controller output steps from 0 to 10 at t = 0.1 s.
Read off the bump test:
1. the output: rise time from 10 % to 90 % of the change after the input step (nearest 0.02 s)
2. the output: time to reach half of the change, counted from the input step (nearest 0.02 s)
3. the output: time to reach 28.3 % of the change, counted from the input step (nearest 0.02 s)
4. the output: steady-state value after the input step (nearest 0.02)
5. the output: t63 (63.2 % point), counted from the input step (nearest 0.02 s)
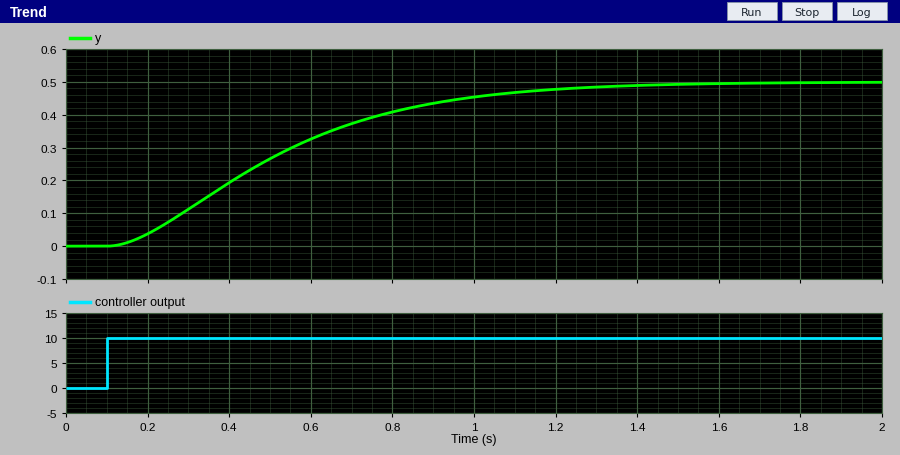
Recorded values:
0.76 s
0.38 s
0.24 s
0.50
0.48 s
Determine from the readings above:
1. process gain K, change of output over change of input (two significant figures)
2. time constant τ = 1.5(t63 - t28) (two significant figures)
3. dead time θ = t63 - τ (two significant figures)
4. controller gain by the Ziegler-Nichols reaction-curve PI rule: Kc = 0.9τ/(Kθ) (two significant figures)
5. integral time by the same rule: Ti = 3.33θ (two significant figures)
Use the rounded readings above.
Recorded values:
0.050
0.36 s
0.12 s
54
0.40 s
